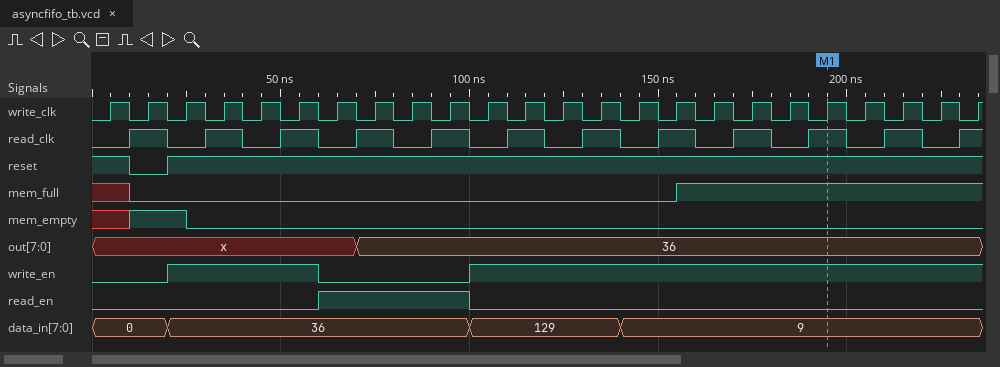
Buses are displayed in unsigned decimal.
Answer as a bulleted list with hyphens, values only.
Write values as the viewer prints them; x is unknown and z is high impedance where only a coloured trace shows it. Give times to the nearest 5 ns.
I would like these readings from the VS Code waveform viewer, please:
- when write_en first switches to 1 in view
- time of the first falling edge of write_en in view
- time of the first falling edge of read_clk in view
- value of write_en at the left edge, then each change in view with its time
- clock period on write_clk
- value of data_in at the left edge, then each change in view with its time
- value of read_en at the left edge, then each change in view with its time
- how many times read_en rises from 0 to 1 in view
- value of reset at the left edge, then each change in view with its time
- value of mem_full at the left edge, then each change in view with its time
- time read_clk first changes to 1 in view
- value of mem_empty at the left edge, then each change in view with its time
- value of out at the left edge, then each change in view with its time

- 20 ns
- 60 ns
- 20 ns
- 0, 1 at 20 ns, 0 at 60 ns, 1 at 100 ns
- 10 ns
- 0, 36 at 20 ns, 129 at 100 ns, 9 at 140 ns
- 0, 1 at 60 ns, 0 at 100 ns
- 1
- 1, 0 at 10 ns, 1 at 20 ns
- x, 0 at 10 ns, 1 at 155 ns
- 10 ns
- x, 1 at 10 ns, 0 at 25 ns
- x, 36 at 70 ns
